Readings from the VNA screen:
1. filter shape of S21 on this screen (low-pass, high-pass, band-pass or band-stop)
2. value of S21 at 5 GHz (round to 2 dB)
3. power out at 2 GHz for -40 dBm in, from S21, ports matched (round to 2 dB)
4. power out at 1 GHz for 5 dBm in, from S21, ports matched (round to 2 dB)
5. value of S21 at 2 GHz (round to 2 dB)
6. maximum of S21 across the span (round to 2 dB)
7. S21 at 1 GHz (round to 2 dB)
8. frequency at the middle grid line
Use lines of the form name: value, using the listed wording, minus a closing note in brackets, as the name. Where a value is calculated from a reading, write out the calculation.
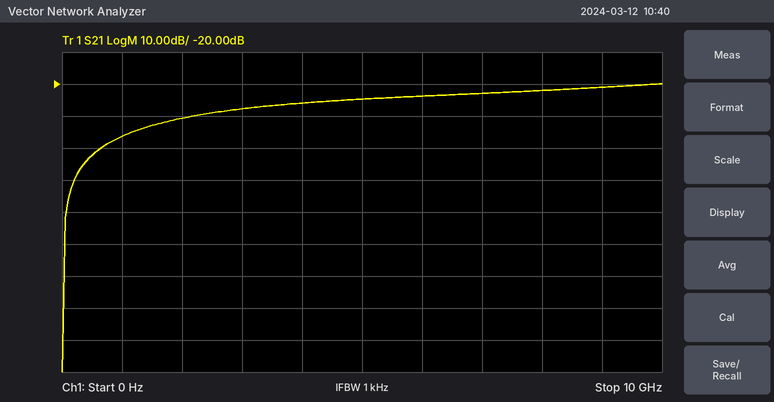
filter shape of S21 on this screen: high-pass
value of S21 at 5 GHz: -24 dB
power out at 2 GHz for -40 dBm in, from S21, ports matched: -40 dBm + (-30 dB) = -70 dBm
power out at 1 GHz for 5 dBm in, from S21, ports matched: 5 dBm + (-36 dB) = -32 dBm
value of S21 at 2 GHz: -30 dB
maximum of S21 across the span: -20 dB
S21 at 1 GHz: -36 dB
frequency at the middle grid line: 5 GHz
